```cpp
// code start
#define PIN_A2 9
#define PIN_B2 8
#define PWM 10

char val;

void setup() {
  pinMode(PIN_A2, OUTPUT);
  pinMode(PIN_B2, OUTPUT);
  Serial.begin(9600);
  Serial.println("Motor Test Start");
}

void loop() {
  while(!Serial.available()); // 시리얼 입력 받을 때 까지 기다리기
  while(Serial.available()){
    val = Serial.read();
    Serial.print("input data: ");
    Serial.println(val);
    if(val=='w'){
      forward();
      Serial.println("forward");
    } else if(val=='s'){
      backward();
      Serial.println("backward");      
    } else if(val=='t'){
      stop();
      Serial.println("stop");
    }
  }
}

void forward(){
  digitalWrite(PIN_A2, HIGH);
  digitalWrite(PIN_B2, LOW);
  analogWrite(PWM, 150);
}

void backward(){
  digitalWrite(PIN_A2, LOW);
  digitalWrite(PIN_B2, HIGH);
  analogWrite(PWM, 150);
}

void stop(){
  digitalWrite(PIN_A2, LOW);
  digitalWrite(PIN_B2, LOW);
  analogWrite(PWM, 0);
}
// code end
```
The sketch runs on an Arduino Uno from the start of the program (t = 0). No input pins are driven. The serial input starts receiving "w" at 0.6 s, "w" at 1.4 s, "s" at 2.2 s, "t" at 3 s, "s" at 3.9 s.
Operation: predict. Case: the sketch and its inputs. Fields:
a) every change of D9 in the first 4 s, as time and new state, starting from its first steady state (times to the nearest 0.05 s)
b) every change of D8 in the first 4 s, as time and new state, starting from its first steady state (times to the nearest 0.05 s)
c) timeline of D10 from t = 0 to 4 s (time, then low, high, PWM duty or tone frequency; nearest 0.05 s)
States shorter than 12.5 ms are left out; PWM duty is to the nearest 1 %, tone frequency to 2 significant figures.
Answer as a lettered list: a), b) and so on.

a) 0 s low; 0.6 s high; 2.2 s low
b) 0 s low; 2.2 s high; 3 s low; 3.9 s high
c) 0.6 s PWM 59 %; 3 s low; 3.9 s PWM 59 %
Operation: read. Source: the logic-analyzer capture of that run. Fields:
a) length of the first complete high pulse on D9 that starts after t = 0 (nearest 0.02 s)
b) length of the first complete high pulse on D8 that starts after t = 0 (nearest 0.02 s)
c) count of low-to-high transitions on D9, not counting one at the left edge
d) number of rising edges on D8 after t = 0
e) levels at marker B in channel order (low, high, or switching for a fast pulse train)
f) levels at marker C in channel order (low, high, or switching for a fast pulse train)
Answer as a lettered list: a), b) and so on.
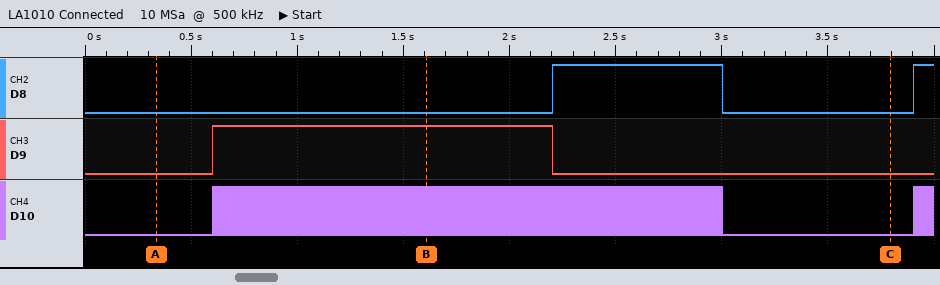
a) 1.60 s
b) 0.80 s
c) 1
d) 2
e) D8 low, D9 high, D10 switching
f) D8 low, D9 low, D10 low
